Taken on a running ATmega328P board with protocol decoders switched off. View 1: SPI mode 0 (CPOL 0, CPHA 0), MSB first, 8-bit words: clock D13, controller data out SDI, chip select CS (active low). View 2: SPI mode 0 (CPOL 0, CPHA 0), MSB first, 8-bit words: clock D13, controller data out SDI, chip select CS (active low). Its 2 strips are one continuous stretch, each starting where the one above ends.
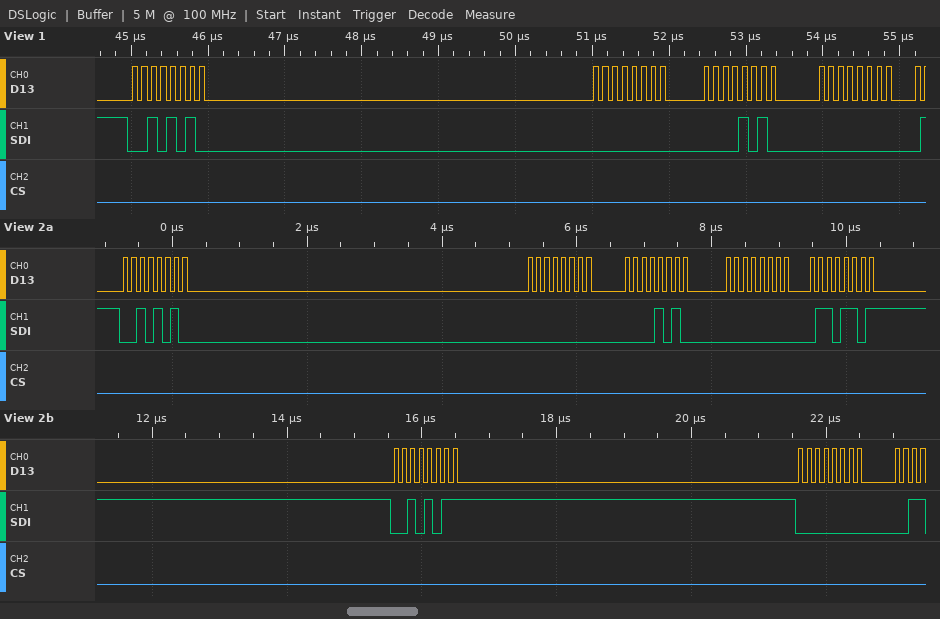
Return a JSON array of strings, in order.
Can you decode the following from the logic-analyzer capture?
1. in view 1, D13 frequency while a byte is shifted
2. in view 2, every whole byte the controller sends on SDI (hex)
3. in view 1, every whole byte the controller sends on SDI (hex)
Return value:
["8 MHz", "2A 00 0A 00 6D 2B 00", "0x2A 0x00 0x0A 0x00"]
